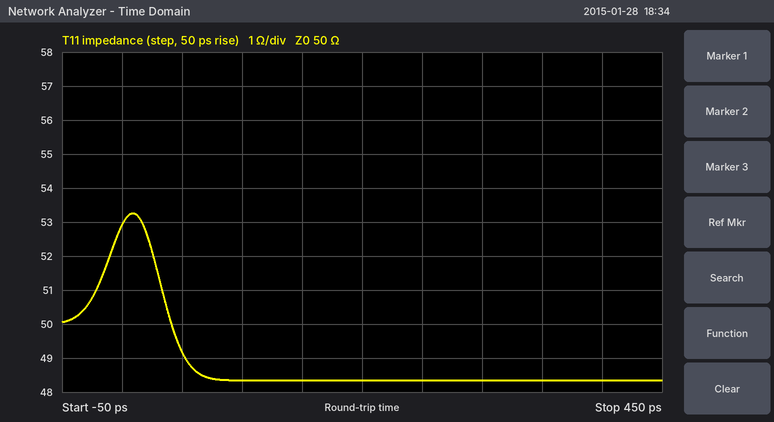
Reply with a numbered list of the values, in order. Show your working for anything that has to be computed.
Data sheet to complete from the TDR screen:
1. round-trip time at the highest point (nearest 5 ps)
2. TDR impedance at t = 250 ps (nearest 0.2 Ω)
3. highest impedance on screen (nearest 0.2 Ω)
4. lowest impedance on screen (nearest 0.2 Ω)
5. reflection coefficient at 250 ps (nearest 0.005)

1. 10 ps
2. 48.4 Ω
3. 53.2 Ω
4. 48.4 Ω
5. (48.4 − 50)/(48.4 + 50) ≈ -0.0163, so -0.015 to the nearest 0.005
